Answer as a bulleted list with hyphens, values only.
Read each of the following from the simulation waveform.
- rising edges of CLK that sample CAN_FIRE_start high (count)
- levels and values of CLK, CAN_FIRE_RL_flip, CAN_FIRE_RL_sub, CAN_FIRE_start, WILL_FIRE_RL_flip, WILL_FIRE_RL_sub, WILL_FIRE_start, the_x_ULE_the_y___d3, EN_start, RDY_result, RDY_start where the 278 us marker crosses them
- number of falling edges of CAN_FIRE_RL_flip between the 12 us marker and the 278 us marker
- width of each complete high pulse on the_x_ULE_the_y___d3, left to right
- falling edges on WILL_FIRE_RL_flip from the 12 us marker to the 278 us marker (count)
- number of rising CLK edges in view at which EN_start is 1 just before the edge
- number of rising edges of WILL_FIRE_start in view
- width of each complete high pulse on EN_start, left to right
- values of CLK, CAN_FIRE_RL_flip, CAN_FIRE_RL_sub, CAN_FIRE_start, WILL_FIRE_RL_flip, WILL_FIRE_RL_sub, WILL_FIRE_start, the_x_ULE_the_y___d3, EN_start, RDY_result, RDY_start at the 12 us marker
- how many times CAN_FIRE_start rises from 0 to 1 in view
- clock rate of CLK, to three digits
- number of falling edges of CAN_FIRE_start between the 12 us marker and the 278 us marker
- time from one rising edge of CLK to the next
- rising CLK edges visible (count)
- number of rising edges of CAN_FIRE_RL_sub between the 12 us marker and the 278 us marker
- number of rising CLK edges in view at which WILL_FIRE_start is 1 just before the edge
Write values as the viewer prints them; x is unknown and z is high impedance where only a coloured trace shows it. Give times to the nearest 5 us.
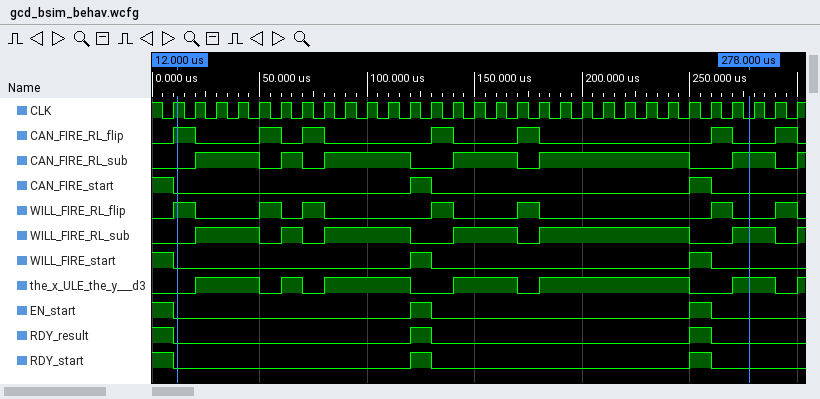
- 3
- CLK=0, CAN_FIRE_RL_flip=0, CAN_FIRE_RL_sub=1, CAN_FIRE_start=0, WILL_FIRE_RL_flip=0, WILL_FIRE_RL_sub=1, WILL_FIRE_start=0, the_x_ULE_the_y___d3=1, EN_start=0, RDY_result=0, RDY_start=0
- 6
- 30 us, 10 us, 40 us, 30 us, 70 us, 20 us
- 6
- 3
- 2
- 10 us, 10 us
- CLK=1, CAN_FIRE_RL_flip=1, CAN_FIRE_RL_sub=0, CAN_FIRE_start=0, WILL_FIRE_RL_flip=1, WILL_FIRE_RL_sub=0, WILL_FIRE_start=0, the_x_ULE_the_y___d3=0, EN_start=0, RDY_result=0, RDY_start=0
- 2
- 100 kHz
- 2
- 10 us
- 30
- 6
- 3
